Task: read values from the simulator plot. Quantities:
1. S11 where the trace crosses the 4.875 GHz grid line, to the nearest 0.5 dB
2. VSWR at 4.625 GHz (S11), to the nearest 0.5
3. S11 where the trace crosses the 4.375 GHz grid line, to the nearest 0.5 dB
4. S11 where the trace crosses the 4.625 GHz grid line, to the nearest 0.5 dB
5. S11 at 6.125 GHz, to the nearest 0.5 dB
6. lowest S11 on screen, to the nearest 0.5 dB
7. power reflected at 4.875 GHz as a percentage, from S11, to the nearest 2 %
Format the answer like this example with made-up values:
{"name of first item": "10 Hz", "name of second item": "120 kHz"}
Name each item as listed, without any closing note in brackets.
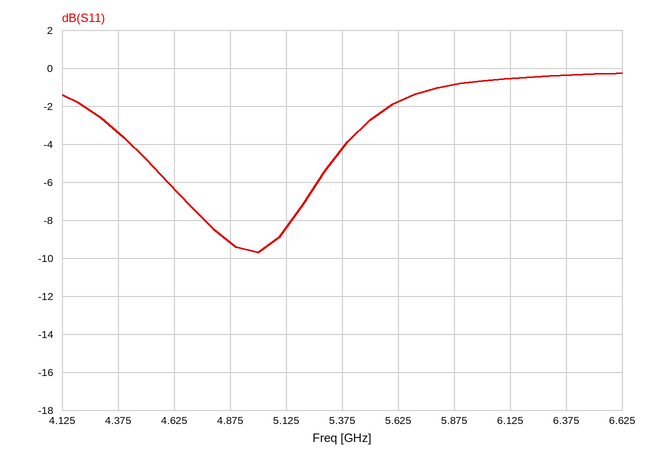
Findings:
{"S11 where the trace crosses the 4.875 GHz grid line, to the nearest 0.5 dB": "-9.0 dB", "VSWR at 4.625 GHz (S11), to the nearest 0.5": "3.0", "S11 where the trace crosses the 4.375 GHz grid line, to the nearest 0.5 dB": "-3.5 dB", "S11 where the trace crosses the 4.625 GHz grid line, to the nearest 0.5 dB": "-6.5 dB", "S11 at 6.125 GHz, to the nearest 0.5 dB": "-0.5 dB", "lowest S11 on screen, to the nearest 0.5 dB": "-9.5 dB", "power reflected at 4.875 GHz as a percentage, from S11, to the nearest 2 %": "12 %"}
